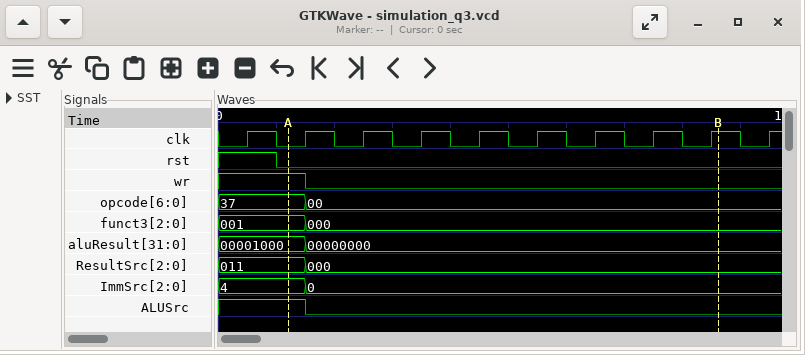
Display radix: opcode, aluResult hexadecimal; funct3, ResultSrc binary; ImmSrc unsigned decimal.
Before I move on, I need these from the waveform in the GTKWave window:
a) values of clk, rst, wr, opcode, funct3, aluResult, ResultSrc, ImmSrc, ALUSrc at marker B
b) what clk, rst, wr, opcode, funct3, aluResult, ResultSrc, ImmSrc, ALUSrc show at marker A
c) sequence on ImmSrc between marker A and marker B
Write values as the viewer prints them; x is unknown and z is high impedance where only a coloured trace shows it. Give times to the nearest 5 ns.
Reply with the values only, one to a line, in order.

clk=1, rst=0, wr=0, opcode=00, funct3=000, aluResult=00000000, ResultSrc=000, ImmSrc=0, ALUSrc=0
clk=0, rst=0, wr=1, opcode=37, funct3=001, aluResult=00001000, ResultSrc=011, ImmSrc=4, ALUSrc=1
4, 0
